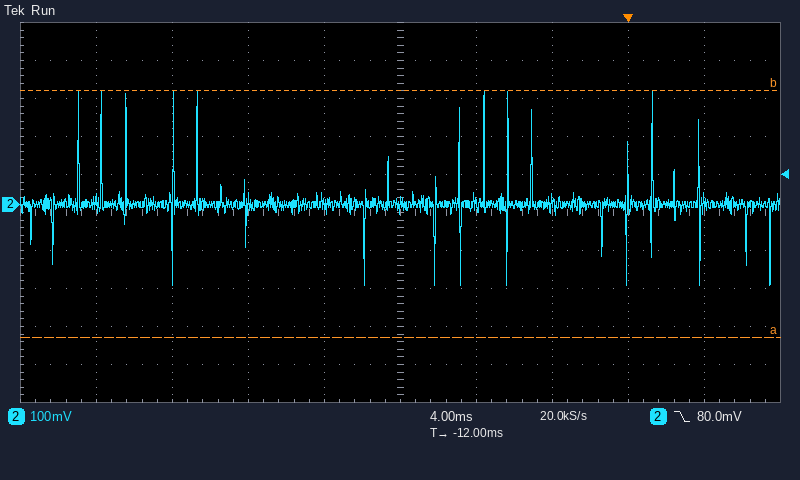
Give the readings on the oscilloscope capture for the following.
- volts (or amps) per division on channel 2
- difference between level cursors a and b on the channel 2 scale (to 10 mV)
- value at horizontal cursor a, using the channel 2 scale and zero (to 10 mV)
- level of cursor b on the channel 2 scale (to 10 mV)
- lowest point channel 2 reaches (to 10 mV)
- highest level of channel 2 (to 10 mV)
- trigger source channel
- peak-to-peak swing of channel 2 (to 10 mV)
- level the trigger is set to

100 mV
650 mV
-350 mV
300 mV
-210 mV
300 mV
channel 2
510 mV
80.0 mV
